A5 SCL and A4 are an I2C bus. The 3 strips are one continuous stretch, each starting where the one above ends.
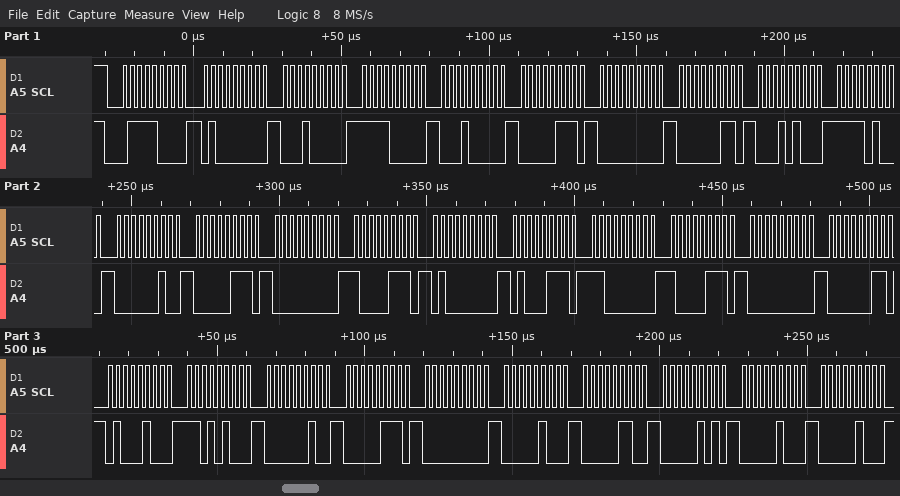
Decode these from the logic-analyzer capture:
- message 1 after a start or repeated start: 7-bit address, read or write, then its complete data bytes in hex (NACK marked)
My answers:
0x3C write: 40 10 F0 10 07 00 03 14 F4 02 07 00 87 40 47 C0 87 00 03 44 D4 02 07 00 04 06 05 04 04
